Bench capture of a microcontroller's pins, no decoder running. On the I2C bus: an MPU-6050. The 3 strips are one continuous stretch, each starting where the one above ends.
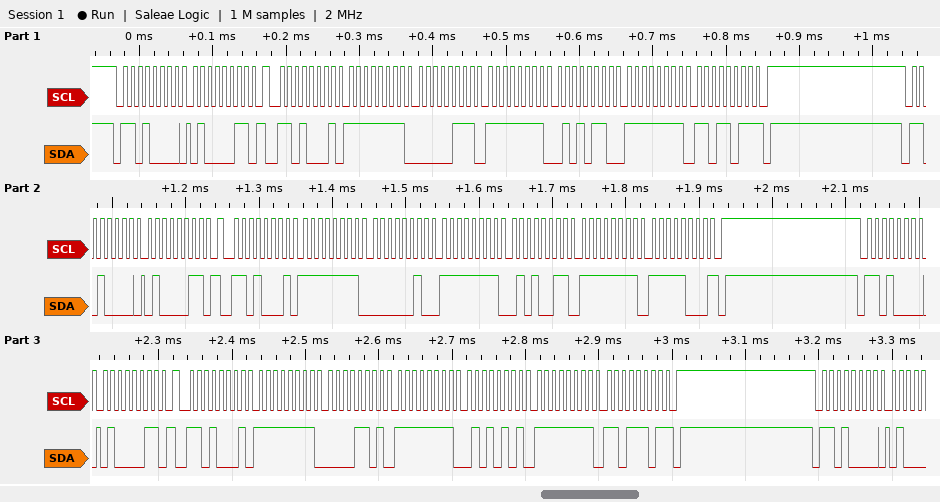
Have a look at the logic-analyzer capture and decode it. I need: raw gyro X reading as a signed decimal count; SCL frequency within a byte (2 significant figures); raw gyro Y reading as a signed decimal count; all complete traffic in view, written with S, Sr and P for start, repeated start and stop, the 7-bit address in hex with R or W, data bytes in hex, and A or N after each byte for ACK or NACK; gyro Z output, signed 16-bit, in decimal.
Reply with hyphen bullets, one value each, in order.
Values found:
- -249
- 100 kHz
- -170
- S 68W A 43 A Sr 68R A FF A 07 A FF A 56 A FF A DB N P S 68W A 43 A Sr 68R A FF A 02 A FF A 53 A FF A F8 N P S 68W A 43 A Sr 68R A FF A 0D A FF A 55 A FF A DD N P S 68W A
- -37
